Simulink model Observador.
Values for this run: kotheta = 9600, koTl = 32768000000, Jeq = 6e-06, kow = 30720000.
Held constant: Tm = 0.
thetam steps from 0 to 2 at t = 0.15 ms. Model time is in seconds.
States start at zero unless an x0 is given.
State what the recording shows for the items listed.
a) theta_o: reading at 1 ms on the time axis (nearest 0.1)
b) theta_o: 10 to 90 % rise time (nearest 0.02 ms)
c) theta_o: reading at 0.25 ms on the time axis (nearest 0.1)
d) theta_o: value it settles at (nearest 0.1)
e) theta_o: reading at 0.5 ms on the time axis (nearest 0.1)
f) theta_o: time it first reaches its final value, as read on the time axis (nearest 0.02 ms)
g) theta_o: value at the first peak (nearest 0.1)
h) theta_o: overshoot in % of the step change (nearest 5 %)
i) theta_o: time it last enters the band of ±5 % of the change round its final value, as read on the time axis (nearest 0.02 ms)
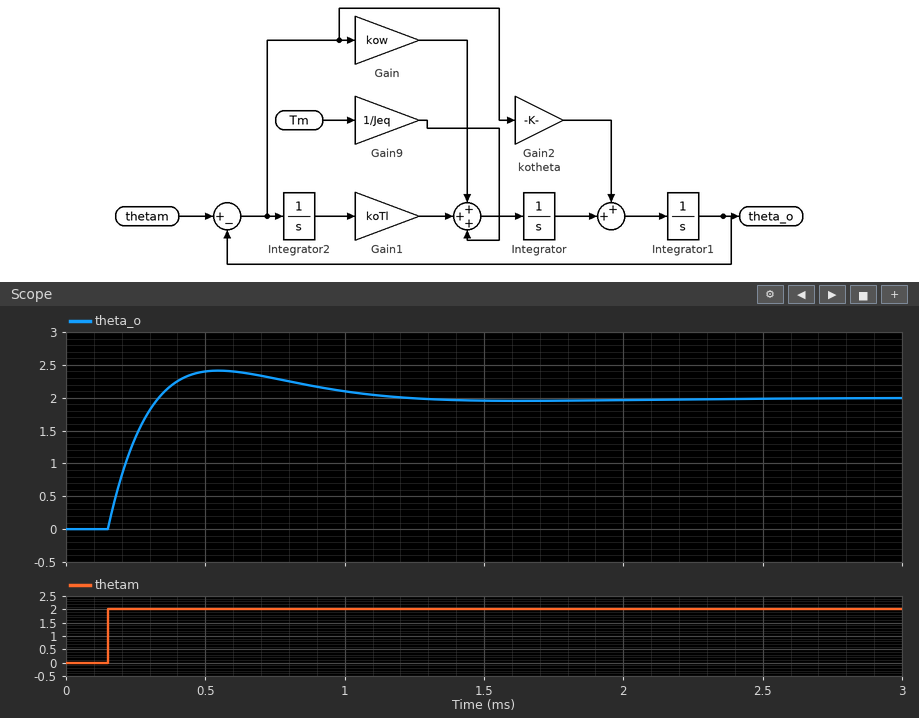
2.1
0.14 ms
1.4
2.0
2.4
0.34 ms
2.4
20 %
1.00 ms
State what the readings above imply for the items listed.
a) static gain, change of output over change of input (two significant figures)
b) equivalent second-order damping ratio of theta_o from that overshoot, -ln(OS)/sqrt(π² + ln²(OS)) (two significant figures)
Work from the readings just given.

1.0
0.46
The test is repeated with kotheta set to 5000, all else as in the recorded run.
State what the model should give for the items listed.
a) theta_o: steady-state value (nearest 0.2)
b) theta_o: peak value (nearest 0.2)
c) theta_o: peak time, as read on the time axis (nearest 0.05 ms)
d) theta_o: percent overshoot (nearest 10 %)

2.0
2.8
0.60 ms
40 %
